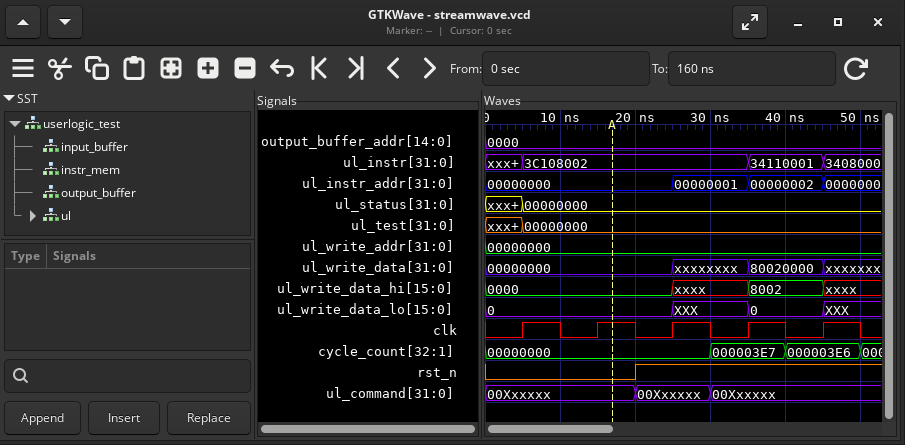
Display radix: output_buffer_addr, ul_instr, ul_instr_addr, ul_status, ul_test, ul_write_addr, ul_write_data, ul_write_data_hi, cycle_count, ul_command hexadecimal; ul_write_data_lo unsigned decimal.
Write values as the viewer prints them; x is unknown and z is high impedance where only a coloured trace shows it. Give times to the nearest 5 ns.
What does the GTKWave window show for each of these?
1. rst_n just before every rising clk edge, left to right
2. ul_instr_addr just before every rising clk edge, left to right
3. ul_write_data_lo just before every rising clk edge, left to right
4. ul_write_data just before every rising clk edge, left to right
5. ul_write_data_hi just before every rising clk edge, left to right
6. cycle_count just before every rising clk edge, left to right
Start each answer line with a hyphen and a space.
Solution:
- 0 0 1 1 1
- 00000000, 00000000, 00000000, 00000001, 00000002
- 0, 0, 0, XXX, 0
- 00000000, 00000000, 00000000, xxxxxxxx, 80020000
- 0000, 0000, 0000, xxxx, 8002
- 00000000, 00000000, 00000000, 000003E7, 000003E6
